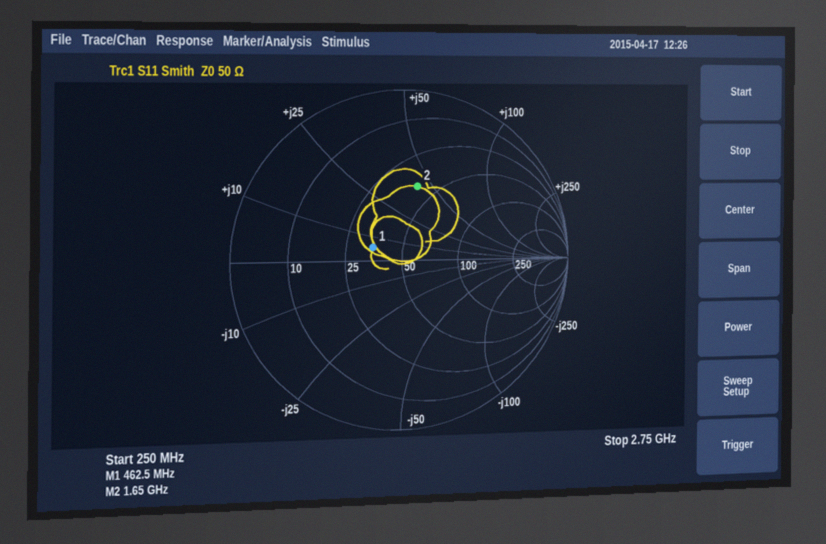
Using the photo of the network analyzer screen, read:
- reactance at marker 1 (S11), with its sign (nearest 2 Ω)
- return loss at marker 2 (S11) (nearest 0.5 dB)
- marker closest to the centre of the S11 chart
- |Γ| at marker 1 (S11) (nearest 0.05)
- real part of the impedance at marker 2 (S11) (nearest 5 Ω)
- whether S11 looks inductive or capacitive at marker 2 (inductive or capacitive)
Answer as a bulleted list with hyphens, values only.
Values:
- +6 Ω
- 7.0 dB
- marker 1
- 0.20
- 40 Ω
- inductive
